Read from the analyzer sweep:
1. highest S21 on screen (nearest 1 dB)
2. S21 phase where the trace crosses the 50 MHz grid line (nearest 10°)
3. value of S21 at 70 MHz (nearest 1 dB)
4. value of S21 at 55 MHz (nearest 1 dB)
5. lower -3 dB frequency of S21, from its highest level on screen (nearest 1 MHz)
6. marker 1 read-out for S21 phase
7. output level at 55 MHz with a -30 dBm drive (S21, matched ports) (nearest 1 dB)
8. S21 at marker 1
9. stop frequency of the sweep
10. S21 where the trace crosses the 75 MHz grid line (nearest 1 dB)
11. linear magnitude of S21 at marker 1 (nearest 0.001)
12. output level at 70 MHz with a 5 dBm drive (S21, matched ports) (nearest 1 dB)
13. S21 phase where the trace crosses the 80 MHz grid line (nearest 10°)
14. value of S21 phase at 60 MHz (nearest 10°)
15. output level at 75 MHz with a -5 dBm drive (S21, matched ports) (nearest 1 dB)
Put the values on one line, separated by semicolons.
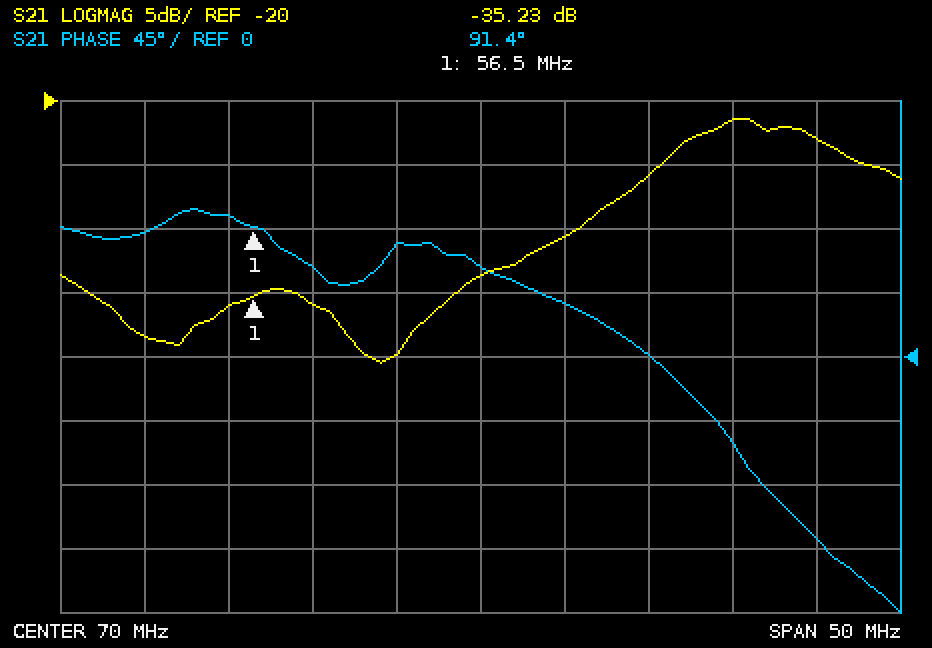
-21 dB; 90°; -34 dB; -36 dB; 81 MHz; 91.4°; -66 dBm; -35.23 dB; 95 MHz; -31 dB; 0.017; -29 dBm; 0°; 60°; -36 dBm
